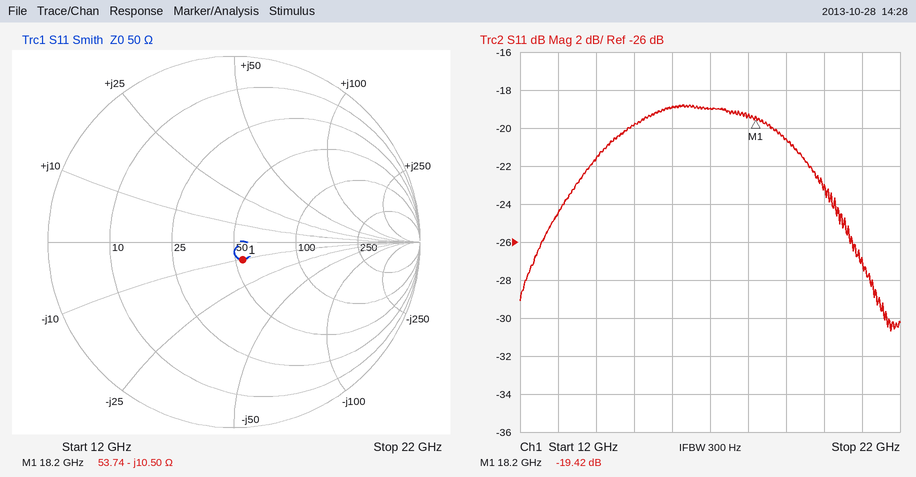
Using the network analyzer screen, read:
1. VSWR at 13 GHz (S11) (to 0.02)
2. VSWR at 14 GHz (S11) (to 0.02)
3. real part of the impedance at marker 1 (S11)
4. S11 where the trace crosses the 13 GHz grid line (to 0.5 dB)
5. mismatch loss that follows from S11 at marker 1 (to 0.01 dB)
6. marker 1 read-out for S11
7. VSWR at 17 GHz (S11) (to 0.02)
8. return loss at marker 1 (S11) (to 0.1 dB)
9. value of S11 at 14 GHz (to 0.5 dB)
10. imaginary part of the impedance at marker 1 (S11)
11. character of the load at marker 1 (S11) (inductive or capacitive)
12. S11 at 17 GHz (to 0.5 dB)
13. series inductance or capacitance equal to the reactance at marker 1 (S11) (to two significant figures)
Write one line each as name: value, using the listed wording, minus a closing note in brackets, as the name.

VSWR at 13 GHz (S11): 1.12
VSWR at 14 GHz (S11): 1.18
real part of the impedance at marker 1: 53.74 Ω
S11 where the trace crosses the 13 GHz grid line: -24.5 dB
mismatch loss that follows from S11 at marker 1: 0.05 dB
marker 1 read-out for S11: -19.42 dB
VSWR at 17 GHz (S11): 1.26
return loss at marker 1 (S11): 19.4 dB
value of S11 at 14 GHz: -21.5 dB
imaginary part of the impedance at marker 1: -10.50 Ω
character of the load at marker 1 (S11): capacitive
S11 at 17 GHz: -19.0 dB
series inductance or capacitance equal to the reactance at marker 1 (S11): 830 fF
